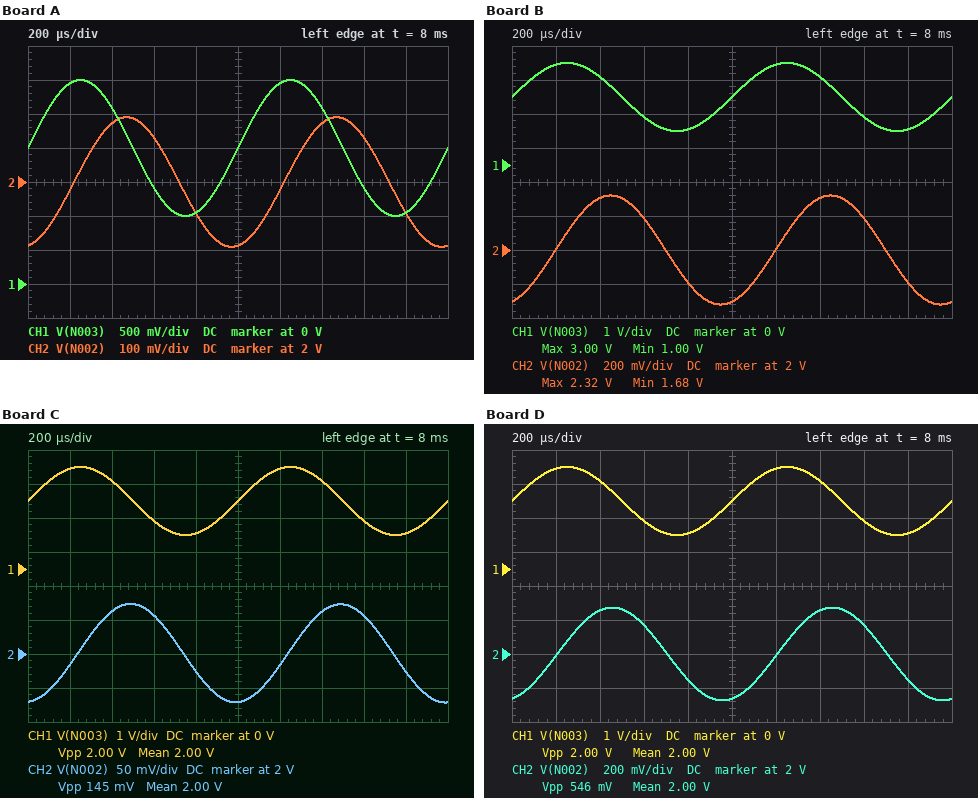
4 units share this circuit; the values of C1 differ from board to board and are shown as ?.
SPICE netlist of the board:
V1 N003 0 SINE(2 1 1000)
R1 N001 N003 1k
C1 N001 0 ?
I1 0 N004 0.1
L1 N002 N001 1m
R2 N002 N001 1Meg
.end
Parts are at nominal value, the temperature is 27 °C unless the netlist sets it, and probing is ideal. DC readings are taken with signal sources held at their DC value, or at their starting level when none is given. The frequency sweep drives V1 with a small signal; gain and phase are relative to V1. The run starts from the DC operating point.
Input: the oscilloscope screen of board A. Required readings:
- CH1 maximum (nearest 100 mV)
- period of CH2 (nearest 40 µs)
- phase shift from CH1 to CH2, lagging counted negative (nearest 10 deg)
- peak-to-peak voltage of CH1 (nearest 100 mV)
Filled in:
3.0 V
1.00 ms
-80 deg
2.0 V
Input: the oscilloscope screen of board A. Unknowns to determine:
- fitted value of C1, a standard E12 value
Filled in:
820 nF
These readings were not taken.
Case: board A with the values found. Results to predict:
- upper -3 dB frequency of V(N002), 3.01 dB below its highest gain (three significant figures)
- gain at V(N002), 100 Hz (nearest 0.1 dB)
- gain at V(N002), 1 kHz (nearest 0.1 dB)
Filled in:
194 Hz
-1.0 dB
-14.4 dB
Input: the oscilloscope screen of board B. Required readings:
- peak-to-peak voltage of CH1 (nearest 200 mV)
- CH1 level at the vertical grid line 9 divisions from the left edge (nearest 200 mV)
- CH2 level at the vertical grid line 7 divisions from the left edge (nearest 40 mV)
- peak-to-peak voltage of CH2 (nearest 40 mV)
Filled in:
2.0 V
1.0 V
2.32 V
640 mV
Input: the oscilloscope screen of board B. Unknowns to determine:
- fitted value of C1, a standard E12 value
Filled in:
470 nF
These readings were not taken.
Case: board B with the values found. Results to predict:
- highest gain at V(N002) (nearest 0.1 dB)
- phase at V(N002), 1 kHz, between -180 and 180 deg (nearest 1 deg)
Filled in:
0 dB
-71 deg
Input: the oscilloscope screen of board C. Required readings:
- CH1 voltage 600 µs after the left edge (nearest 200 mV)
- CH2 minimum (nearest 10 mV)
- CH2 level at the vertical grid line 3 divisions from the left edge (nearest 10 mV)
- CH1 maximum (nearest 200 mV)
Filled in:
1.4 V
1.93 V
2.06 V
3.0 V
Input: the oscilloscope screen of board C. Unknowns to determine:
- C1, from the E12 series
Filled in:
2.2 µF
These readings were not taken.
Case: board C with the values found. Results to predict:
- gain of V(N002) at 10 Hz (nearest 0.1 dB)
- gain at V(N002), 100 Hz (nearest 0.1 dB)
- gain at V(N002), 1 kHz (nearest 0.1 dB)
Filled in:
-0.1 dB
-4.6 dB
-22.8 dB
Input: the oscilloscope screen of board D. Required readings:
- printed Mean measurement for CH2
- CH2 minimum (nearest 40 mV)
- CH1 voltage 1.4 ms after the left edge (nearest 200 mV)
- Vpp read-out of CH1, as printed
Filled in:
2.00 V
1.72 V
2.6 V
2.00 V
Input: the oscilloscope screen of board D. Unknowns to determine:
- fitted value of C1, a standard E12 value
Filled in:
560 nF
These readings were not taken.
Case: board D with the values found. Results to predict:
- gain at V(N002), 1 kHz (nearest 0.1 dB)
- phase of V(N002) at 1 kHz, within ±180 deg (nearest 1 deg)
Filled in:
-11.3 dB
-74 deg
